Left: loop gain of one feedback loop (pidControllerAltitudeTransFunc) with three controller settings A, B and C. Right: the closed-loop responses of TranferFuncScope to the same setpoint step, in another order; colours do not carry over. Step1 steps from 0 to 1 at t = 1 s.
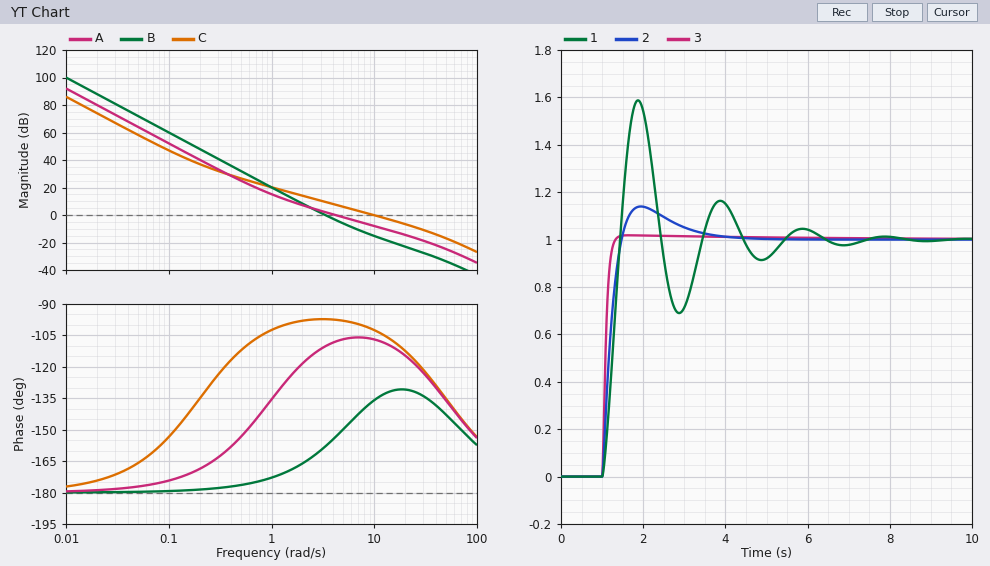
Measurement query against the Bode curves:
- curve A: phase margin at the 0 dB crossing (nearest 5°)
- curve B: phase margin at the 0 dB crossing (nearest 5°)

70°
20°
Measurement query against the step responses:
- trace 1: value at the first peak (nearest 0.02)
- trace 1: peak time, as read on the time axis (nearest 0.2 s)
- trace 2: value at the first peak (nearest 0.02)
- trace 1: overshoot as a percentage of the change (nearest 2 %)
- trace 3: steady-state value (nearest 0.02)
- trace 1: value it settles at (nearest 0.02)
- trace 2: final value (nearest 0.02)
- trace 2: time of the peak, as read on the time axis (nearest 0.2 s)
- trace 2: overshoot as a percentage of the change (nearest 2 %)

1.58
1.8 s
1.14
58 %
1.00
1.00
1.00
2.0 s
14 %
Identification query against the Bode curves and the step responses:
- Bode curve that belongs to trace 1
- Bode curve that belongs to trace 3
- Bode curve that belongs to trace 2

B
C
A
